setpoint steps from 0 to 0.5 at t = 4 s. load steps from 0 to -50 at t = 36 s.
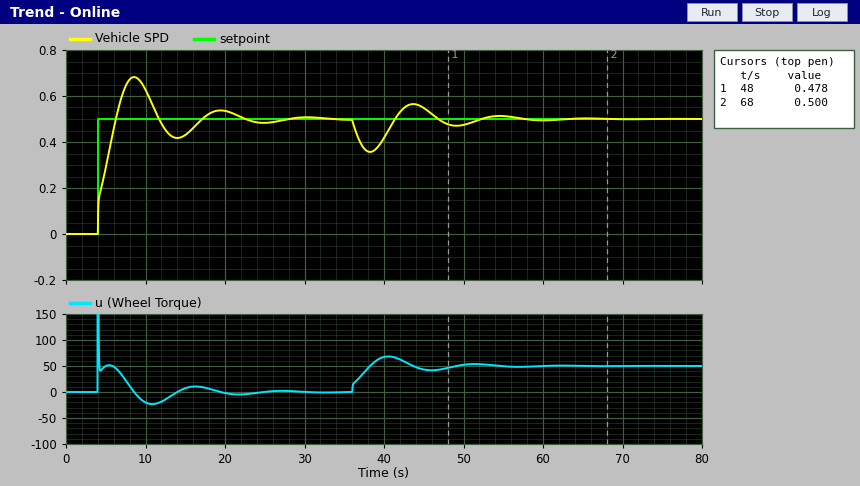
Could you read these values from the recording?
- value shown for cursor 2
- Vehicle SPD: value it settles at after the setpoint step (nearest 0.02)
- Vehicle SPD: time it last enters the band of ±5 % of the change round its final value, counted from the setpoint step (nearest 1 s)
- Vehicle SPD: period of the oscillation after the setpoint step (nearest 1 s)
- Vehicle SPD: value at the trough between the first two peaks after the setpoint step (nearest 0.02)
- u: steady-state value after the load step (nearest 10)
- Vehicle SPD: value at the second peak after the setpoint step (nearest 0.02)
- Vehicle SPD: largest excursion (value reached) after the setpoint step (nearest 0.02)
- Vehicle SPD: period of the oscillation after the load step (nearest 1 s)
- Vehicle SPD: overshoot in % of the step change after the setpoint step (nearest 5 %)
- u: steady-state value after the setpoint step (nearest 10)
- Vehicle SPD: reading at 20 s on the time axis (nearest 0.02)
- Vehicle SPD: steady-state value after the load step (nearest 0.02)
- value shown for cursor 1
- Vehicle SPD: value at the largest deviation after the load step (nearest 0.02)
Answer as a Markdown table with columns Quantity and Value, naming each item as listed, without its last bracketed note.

| Quantity | Value |
|---|---|
| value shown for cursor 2 | 0.500 |
| Vehicle SPD: value it settles at after the setpoint step | 0.50 |
| Vehicle SPD: time it last enters the band of ±5 % of the change round its final value, counted from the setpoint step | 17 s |
| Vehicle SPD: period of the oscillation after the setpoint step | 11 s |
| Vehicle SPD: value at the trough between the first two peaks after the setpoint step | 0.42 |
| u: steady-state value after the load step | 50 |
| Vehicle SPD: value at the second peak after the setpoint step | 0.54 |
| Vehicle SPD: largest excursion (value reached) after the setpoint step | 0.68 |
| Vehicle SPD: period of the oscillation after the load step | 11 s |
| Vehicle SPD: overshoot in % of the step change after the setpoint step | 35 % |
| u: steady-state value after the setpoint step | 0 |
| Vehicle SPD: reading at 20 s on the time axis | 0.54 |
| Vehicle SPD: steady-state value after the load step | 0.50 |
| value shown for cursor 1 | 0.478 |
| Vehicle SPD: value at the largest deviation after the load step | 0.36 |
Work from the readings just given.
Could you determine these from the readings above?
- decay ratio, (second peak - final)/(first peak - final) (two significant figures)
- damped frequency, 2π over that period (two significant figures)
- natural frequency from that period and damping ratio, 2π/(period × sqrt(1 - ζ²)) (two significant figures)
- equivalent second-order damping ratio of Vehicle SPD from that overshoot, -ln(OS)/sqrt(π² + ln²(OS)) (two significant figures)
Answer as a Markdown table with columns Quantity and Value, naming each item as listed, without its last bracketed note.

| Quantity | Value |
|---|---|
| decay ratio, (second peak - final)/(first peak - final) | 0.22 |
| damped frequency, 2π over that period | 0.57 rad/s |
| natural frequency from that period and damping ratio, 2π/(period × sqrt(1 - ζ²)) | 0.60 rad/s |
| equivalent second-order damping ratio of Vehicle SPD from that overshoot, -ln(OS)/sqrt(π² + ln²(OS)) | 0.32 |
